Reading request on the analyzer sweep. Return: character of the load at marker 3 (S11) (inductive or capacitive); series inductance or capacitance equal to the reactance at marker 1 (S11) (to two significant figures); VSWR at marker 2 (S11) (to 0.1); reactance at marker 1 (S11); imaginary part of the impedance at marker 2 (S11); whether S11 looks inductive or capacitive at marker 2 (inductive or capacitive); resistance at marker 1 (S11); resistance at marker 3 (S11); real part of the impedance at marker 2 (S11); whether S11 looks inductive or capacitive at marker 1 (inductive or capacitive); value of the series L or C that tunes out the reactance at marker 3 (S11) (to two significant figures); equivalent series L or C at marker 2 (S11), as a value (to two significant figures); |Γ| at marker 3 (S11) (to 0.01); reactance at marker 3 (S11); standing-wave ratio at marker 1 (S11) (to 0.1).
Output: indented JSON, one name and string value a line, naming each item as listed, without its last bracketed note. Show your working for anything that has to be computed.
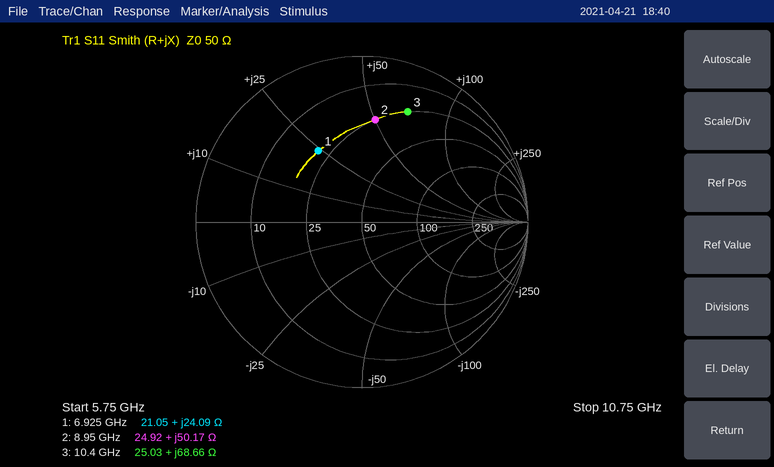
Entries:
{
  "character of the load at marker 3 (S11)": "inductive",
  "series inductance or capacitance equal to the reactance at marker 1 (S11)": "L = 24.09 Ω/(2π × 6.925 GHz) ≈ 554 pH, so 550 pH to two significant figures",
  "VSWR at marker 2 (S11)": "4.3",
  "reactance at marker 1": "+24.09 Ω",
  "imaginary part of the impedance at marker 2": "+50.17 Ω",
  "whether S11 looks inductive or capacitive at marker 2": "inductive",
  "resistance at marker 1": "21.05 Ω",
  "resistance at marker 3": "25.03 Ω",
  "real part of the impedance at marker 2": "24.92 Ω",
  "whether S11 looks inductive or capacitive at marker 1": "inductive",
  "value of the series L or C that tunes out the reactance at marker 3 (S11)": "C = 1/(2π × 10.4 GHz × 68.66 Ω) ≈ 223 fF, so 220 fF to two significant figures",
  "equivalent series L or C at marker 2 (S11), as a value": "L = 50.17 Ω/(2π × 8.95 GHz) ≈ 892 pH, so 890 pH to two significant figures",
  "|Γ| at marker 3 (S11)": "0.72",
  "reactance at marker 3": "+68.66 Ω",
  "standing-wave ratio at marker 1 (S11)": "3.0"
}
